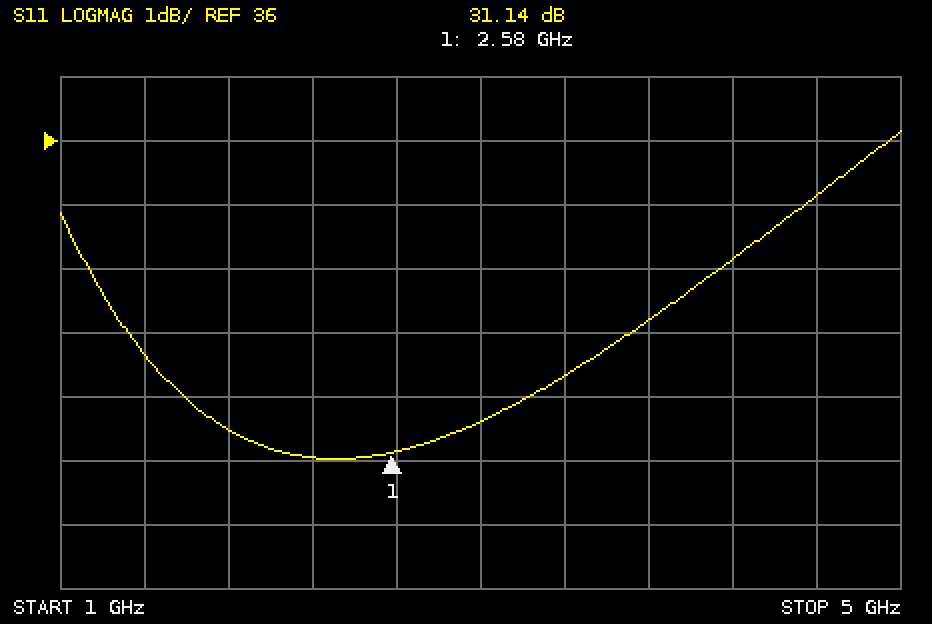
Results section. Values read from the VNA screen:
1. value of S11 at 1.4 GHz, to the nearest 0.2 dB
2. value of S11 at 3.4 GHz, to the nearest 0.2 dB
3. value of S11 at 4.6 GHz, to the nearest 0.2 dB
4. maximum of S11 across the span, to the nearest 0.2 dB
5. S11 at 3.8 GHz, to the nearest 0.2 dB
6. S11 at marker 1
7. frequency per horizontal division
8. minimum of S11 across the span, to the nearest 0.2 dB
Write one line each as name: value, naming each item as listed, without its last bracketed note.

value of S11 at 1.4 GHz, to the nearest 0.2 dB: 32.6 dB
value of S11 at 3.4 GHz, to the nearest 0.2 dB: 32.4 dB
value of S11 at 4.6 GHz, to the nearest 0.2 dB: 35.2 dB
maximum of S11 across the span, to the nearest 0.2 dB: 36.2 dB
S11 at 3.8 GHz, to the nearest 0.2 dB: 33.2 dB
S11 at marker 1: 31.14 dB
frequency per horizontal division: 400 MHz
minimum of S11 across the span, to the nearest 0.2 dB: 31.0 dB
